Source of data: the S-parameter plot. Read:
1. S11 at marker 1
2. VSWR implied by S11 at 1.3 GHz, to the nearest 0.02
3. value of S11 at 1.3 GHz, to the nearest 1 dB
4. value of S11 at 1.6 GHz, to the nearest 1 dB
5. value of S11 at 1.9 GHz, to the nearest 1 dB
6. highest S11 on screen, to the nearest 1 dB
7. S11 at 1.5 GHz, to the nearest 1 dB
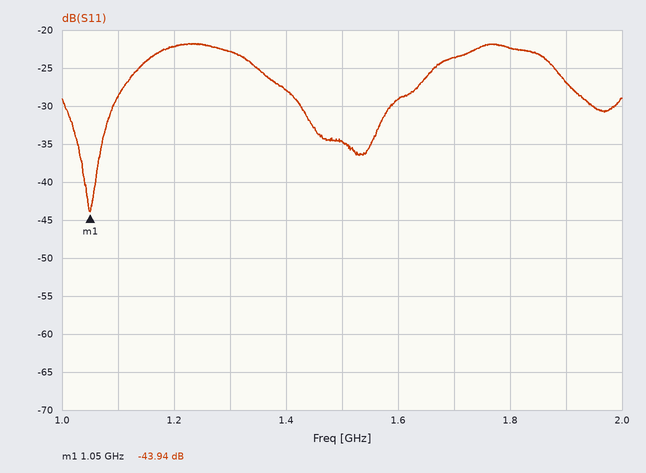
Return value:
-43.94 dB
1.16
-23 dB
-29 dB
-27 dB
-22 dB
-35 dB
